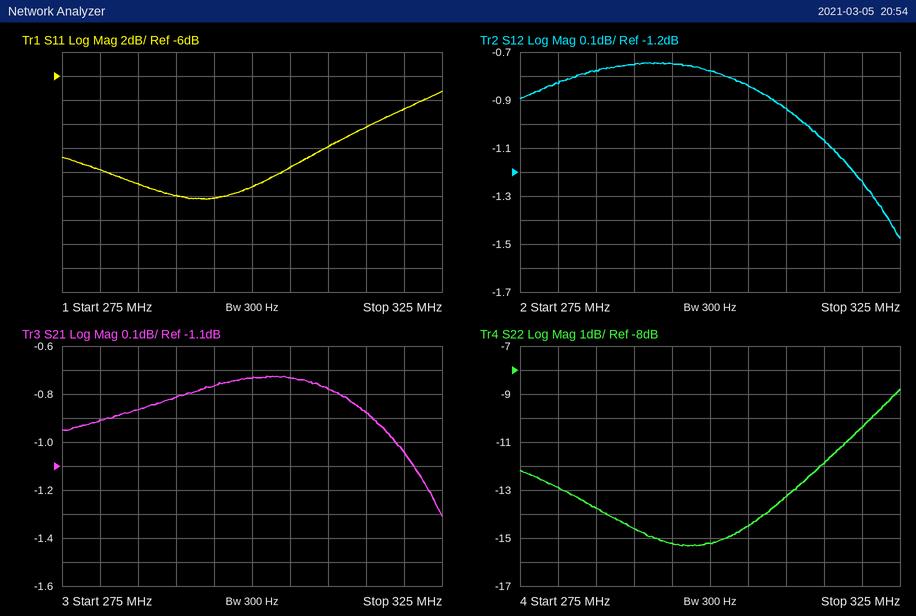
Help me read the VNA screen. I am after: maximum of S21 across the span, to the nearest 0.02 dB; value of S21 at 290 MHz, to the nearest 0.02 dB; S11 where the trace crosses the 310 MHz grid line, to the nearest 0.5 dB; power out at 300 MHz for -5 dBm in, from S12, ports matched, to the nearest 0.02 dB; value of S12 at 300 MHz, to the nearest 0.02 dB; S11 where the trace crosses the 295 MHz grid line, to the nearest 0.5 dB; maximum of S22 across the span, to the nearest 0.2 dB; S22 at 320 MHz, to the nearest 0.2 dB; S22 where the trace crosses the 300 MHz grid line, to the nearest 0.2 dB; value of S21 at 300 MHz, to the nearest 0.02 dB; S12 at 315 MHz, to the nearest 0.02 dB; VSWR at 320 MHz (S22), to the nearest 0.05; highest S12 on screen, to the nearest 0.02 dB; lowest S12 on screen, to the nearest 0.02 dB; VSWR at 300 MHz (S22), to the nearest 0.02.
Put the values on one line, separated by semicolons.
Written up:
-0.72 dB; -0.82 dB; -12.0 dB; -5.78 dBm; -0.78 dB; -16.0 dB; -8.8 dB; -10.4 dB; -15.2 dB; -0.74 dB; -1.06 dB; 1.85; -0.74 dB; -1.48 dB; 1.42
